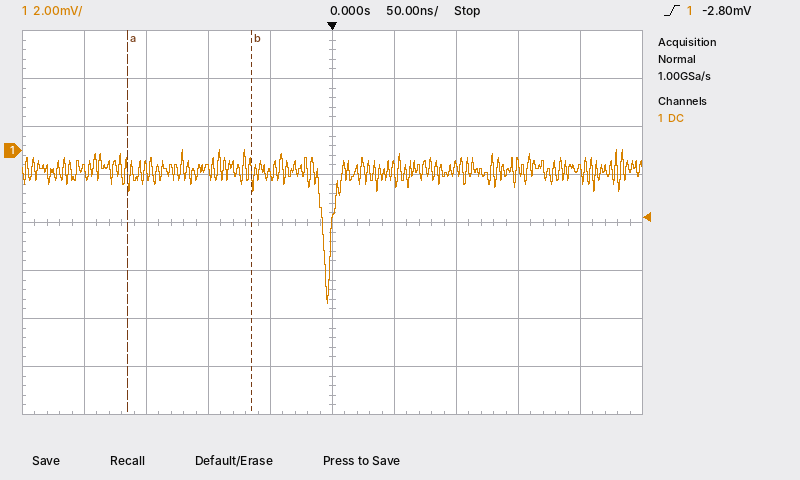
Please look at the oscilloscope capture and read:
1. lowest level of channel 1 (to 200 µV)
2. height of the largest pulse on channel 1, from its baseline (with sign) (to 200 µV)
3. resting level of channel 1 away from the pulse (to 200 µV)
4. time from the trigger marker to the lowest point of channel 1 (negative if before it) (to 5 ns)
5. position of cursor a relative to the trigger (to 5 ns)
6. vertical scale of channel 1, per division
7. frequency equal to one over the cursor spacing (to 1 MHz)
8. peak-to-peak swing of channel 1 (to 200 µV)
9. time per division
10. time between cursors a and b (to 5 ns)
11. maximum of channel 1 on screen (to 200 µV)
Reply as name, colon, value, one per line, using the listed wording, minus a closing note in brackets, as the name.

lowest level of channel 1: -6.4 mV
height of the largest pulse on channel 1, from its baseline (with sign): -5.6 mV
resting level of channel 1 away from the pulse: -800 µV
time from the trigger marker to the lowest point of channel 1 (negative if before it): -5 ns
position of cursor a relative to the trigger: -165 ns
vertical scale of channel 1, per division: 2 mV
frequency equal to one over the cursor spacing: 10 MHz
peak-to-peak swing of channel 1: 6.4 mV
time per division: 50 ns
time between cursors a and b: 100 ns
maximum of channel 1 on screen: 0.0 mV
